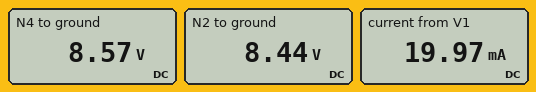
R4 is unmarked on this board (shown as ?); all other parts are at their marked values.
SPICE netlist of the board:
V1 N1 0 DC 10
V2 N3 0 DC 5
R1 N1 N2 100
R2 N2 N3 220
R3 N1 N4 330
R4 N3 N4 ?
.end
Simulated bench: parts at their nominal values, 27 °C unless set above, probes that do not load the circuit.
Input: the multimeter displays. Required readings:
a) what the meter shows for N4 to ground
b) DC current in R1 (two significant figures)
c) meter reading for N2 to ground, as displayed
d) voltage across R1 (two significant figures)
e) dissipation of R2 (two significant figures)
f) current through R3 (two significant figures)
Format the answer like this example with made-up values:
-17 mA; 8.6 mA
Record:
8.57 V; 16 mA; 8.44 V; 1.6 V; 54 mW; 4.3 mA
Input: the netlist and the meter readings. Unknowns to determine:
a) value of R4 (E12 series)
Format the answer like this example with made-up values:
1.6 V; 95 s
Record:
820 Ω
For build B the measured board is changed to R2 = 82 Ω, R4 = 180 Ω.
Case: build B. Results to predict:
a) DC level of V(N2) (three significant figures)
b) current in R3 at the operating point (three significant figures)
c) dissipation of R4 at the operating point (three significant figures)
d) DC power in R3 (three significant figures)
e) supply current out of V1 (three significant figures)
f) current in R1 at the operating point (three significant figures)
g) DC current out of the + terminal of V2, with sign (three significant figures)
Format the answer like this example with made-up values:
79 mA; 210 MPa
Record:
7.25 V; 9.80 mA; 17.3 mW; 31.7 mW; 37.3 mA; 27.5 mA; -37.3 mA
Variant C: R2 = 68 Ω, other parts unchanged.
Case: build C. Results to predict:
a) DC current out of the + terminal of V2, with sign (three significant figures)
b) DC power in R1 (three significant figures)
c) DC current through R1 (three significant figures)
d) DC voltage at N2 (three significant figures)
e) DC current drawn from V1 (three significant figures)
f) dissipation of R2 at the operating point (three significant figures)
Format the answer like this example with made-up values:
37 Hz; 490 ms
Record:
-34.1 mA; 88.6 mW; 29.8 mA; 7.02 V; 34.1 mA; 60.2 mW
